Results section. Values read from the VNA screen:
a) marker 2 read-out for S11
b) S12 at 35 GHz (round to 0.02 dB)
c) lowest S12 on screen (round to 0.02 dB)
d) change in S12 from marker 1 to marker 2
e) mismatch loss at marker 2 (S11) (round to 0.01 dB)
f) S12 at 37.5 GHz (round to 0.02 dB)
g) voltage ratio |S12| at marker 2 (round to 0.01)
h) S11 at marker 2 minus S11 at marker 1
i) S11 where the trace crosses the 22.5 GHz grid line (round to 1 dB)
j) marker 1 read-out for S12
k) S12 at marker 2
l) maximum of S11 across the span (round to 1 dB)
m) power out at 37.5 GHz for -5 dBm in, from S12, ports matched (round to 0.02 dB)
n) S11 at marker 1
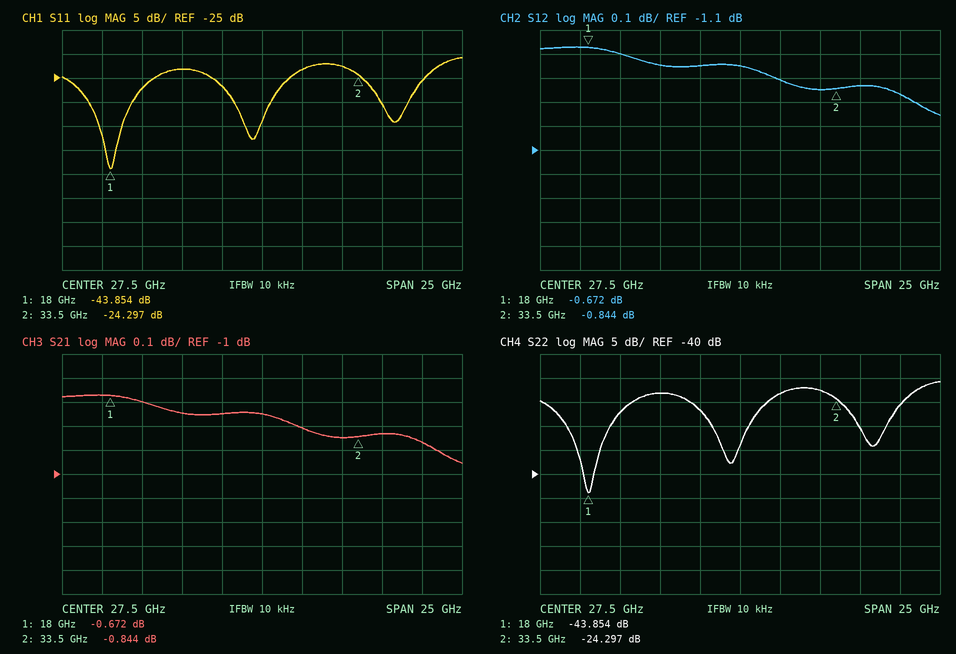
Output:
-24.297 dB
-0.84 dB
-0.96 dB
-0.172 dB
0.02 dB
-0.86 dB
0.91
19.557 dB
-23 dB
-0.672 dB
-0.844 dB
-21 dB
-5.86 dBm
-43.854 dB
